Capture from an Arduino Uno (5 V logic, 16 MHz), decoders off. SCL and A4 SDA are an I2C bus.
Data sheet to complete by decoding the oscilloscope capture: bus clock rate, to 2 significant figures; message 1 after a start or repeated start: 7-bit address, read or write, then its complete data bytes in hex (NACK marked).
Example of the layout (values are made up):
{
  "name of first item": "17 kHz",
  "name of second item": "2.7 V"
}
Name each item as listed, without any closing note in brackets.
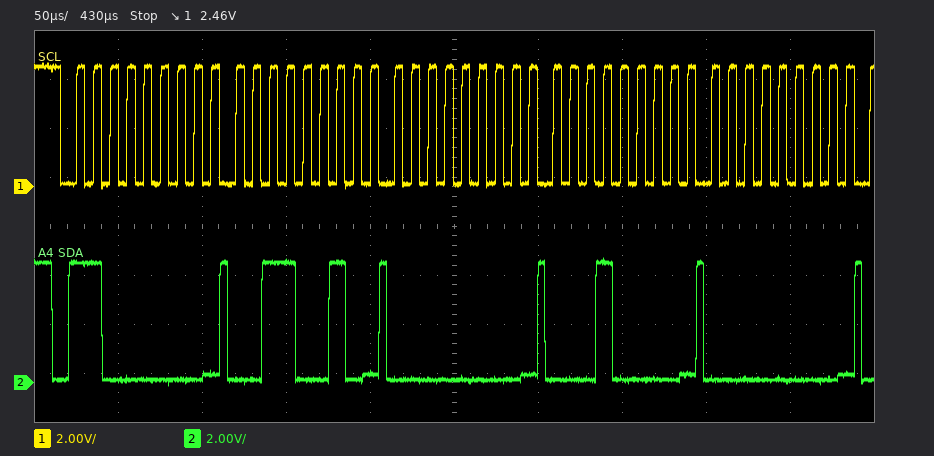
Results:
{
  "bus clock rate, to 2 significant figures": "100 kHz",
  "message 1 after a start or repeated start: 7-bit address, read or write, then its complete data bytes in hex": "0x60 write: 32 00 10 00"
}
